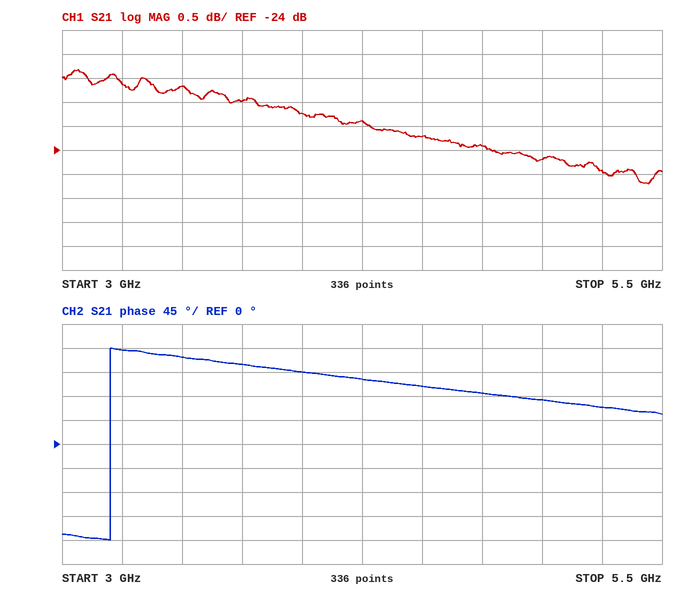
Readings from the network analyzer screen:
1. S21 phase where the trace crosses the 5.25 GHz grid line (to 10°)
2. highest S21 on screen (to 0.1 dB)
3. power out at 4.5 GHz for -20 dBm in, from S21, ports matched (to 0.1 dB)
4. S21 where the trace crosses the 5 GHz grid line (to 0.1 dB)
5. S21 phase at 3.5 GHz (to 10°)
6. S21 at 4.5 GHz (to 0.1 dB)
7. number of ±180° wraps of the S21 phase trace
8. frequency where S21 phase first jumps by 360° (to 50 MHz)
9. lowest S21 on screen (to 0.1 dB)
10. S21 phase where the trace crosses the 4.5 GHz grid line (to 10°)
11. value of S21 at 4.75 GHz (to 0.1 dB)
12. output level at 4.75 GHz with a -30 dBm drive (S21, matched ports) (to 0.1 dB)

70°
-22.3 dB
-43.7 dBm
-24.2 dB
160°
-23.7 dB
1
3.20 GHz
-24.7 dB
110°
-23.9 dB
-53.9 dBm
